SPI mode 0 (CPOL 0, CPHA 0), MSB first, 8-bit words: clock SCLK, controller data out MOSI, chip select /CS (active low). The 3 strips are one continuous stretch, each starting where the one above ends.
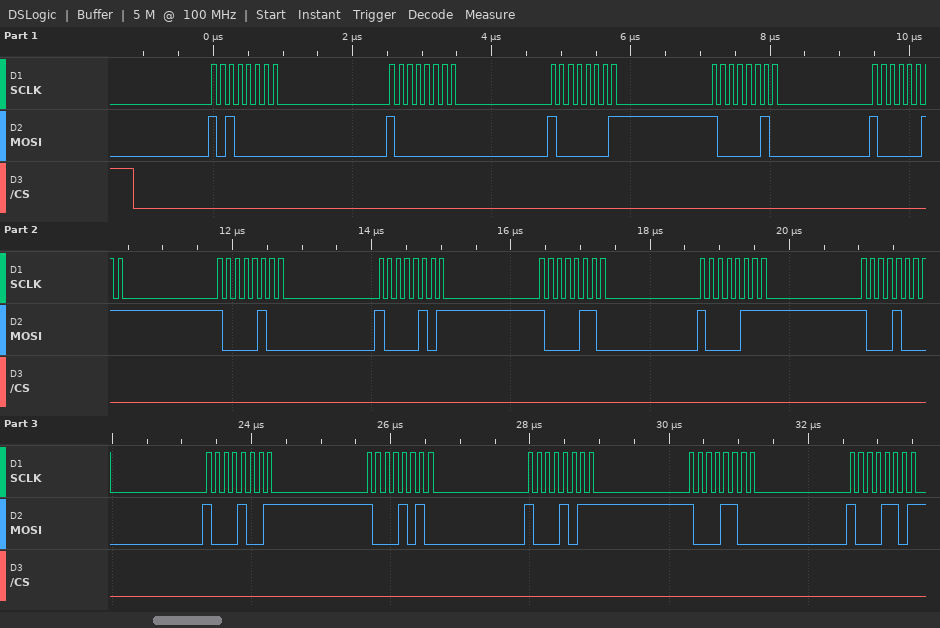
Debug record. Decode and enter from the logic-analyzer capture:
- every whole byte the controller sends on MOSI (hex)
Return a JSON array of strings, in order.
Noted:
["A0 80 81 82 83 84 85 86 87 88 89 8A 8B 8C 8D"]
